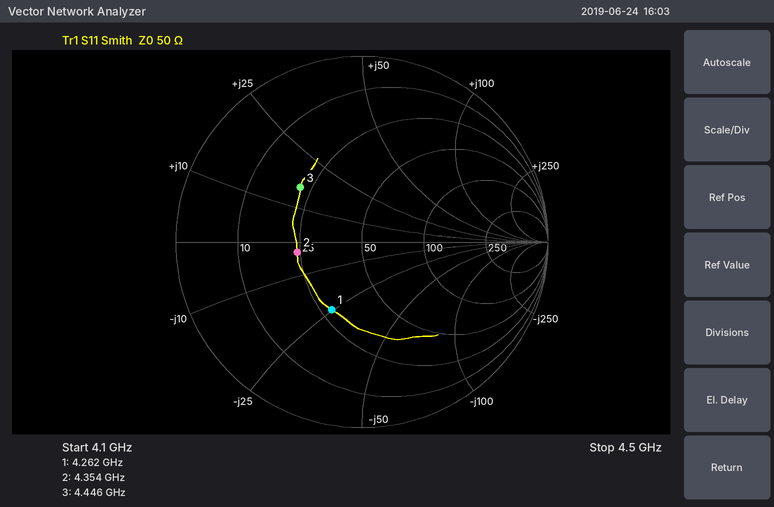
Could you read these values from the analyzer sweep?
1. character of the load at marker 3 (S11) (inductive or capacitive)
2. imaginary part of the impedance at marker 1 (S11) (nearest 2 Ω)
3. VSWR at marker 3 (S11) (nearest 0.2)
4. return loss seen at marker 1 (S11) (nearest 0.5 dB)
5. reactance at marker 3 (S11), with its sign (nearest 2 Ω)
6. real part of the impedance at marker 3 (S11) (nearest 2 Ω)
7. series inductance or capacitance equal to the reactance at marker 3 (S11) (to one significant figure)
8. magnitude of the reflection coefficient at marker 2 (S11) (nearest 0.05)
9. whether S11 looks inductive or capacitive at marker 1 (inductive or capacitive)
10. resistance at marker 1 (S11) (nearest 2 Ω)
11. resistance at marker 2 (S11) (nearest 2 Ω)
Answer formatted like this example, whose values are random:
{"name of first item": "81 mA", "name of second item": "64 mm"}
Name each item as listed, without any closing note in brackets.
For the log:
{"character of the load at marker 3 (S11)": "inductive", "imaginary part of the impedance at marker 1 (S11)": "-24 Ω", "VSWR at marker 3 (S11)": "2.6", "return loss seen at marker 1 (S11)": "8.0 dB", "reactance at marker 3 (S11), with its sign": "+16 Ω", "real part of the impedance at marker 3 (S11)": "22 Ω", "series inductance or capacitance equal to the reactance at marker 3 (S11)": "600 pH", "magnitude of the reflection coefficient at marker 2 (S11)": "0.35", "whether S11 looks inductive or capacitive at marker 1": "capacitive", "resistance at marker 1 (S11)": "28 Ω", "resistance at marker 2 (S11)": "24 Ω"}
